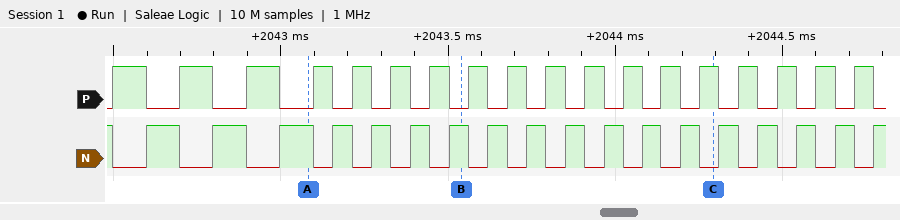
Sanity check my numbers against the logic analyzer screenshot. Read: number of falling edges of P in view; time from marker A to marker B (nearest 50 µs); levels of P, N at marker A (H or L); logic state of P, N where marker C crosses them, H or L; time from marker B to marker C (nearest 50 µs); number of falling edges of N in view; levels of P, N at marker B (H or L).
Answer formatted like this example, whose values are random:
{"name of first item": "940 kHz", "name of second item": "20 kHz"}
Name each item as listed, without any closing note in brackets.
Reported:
{"number of falling edges of P in view": "18", "time from marker A to marker B": "450 µs", "levels of P, N at marker A": "P=L, N=H", "logic state of P, N where marker C crosses them, H or L": "P=H, N=L", "time from marker B to marker C": "750 µs", "number of falling edges of N in view": "18", "levels of P, N at marker B": "P=L, N=H"}
